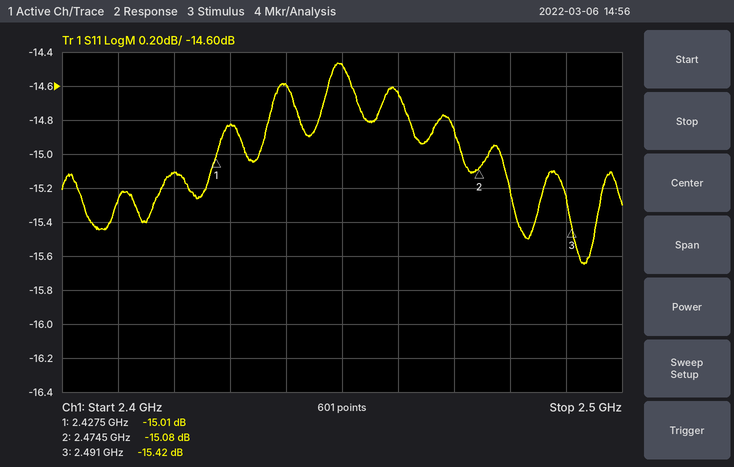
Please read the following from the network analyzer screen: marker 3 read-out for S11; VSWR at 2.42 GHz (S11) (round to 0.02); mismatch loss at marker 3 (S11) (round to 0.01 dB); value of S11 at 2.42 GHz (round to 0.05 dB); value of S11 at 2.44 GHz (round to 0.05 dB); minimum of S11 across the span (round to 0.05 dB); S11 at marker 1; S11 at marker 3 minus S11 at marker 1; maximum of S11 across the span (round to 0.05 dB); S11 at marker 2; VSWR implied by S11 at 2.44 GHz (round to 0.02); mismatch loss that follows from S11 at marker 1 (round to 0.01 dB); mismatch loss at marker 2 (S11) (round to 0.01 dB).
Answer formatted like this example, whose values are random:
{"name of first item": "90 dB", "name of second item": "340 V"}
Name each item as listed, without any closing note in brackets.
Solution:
{"marker 3 read-out for S11": "-15.42 dB", "VSWR at 2.42 GHz (S11)": "1.42", "mismatch loss at marker 3 (S11)": "0.13 dB", "value of S11 at 2.42 GHz": "-15.10 dB", "value of S11 at 2.44 GHz": "-14.60 dB", "minimum of S11 across the span": "-15.65 dB", "S11 at marker 1": "-15.01 dB", "S11 at marker 3 minus S11 at marker 1": "-0.41 dB", "maximum of S11 across the span": "-14.45 dB", "S11 at marker 2": "-15.08 dB", "VSWR implied by S11 at 2.44 GHz": "1.46", "mismatch loss that follows from S11 at marker 1": "0.14 dB", "mismatch loss at marker 2 (S11)": "0.14 dB"}
